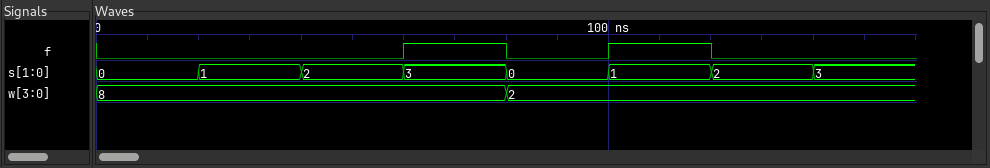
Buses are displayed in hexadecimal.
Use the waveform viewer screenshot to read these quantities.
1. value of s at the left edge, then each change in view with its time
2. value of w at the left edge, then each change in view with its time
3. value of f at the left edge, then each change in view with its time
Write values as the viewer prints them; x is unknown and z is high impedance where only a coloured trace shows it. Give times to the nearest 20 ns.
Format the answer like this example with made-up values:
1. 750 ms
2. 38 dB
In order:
1. 0, 1 at 20 ns, 2 at 40 ns, 3 at 60 ns, 0 at 80 ns, 1 at 100 ns, 2 at 120 ns, 3 at 140 ns
2. 8, 2 at 80 ns
3. 0, 1 at 60 ns, 0 at 80 ns, 1 at 100 ns, 0 at 120 ns
